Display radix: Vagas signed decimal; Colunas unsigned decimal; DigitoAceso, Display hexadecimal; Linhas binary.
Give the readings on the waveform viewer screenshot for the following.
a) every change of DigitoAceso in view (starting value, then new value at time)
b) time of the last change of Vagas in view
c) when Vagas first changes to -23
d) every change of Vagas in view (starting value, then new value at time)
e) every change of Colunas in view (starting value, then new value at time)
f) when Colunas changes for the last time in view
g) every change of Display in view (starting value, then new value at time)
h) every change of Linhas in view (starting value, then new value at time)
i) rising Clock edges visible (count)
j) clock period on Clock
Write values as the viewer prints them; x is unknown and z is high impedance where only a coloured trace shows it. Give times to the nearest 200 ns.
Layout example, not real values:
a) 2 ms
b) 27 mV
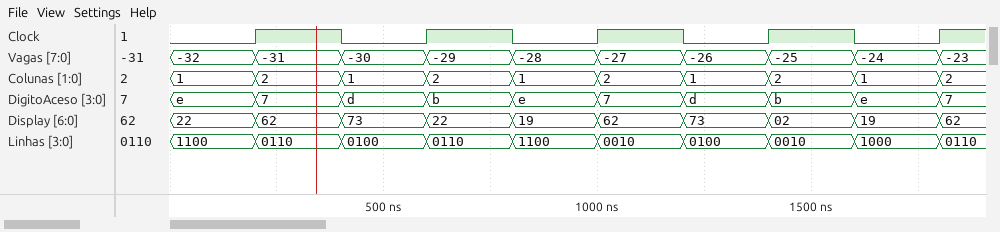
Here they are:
a) e, 7 at 200 ns, d at 400 ns, b at 600 ns, e at 800 ns, 7 at 1000 ns, d at 1200 ns, b at 1400 ns, e at 1600 ns, 7 at 1800 ns
b) 1800 ns
c) 1800 ns
d) -32, -31 at 200 ns, -30 at 400 ns, -29 at 600 ns, -28 at 800 ns, -27 at 1000 ns, -26 at 1200 ns, -25 at 1400 ns, -24 at 1600 ns, -23 at 1800 ns
e) 1, 2 at 200 ns, 1 at 400 ns, 2 at 600 ns, 1 at 800 ns, 2 at 1000 ns, 1 at 1200 ns, 2 at 1400 ns, 1 at 1600 ns, 2 at 1800 ns
f) 1800 ns
g) 22, 62 at 200 ns, 73 at 400 ns, 22 at 600 ns, 19 at 800 ns, 62 at 1000 ns, 73 at 1200 ns, 02 at 1400 ns, 19 at 1600 ns, 62 at 1800 ns
h) 1100, 0110 at 200 ns, 0100 at 400 ns, 0110 at 600 ns, 1100 at 800 ns, 0010 at 1000 ns, 0100 at 1200 ns, 0010 at 1400 ns, 1000 at 1600 ns, 0110 at 1800 ns
i) 5
j) 400 ns
